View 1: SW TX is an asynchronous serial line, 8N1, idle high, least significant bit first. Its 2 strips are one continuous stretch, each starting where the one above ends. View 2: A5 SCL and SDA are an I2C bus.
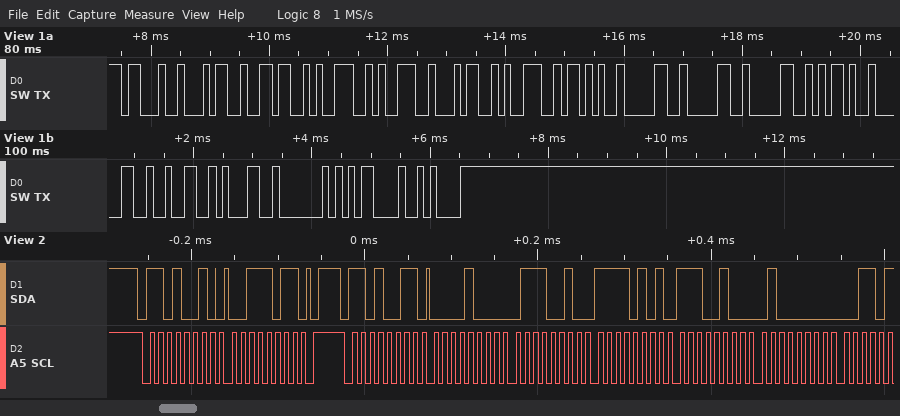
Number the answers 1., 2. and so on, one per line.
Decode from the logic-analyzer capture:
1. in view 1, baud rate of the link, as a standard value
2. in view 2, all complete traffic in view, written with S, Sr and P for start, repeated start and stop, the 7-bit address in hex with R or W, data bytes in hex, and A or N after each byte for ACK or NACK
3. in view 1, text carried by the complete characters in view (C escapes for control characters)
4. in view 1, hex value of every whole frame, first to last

1. 9600 baud
2. S 69W A 3B A P S 69R A 08 A 72 A F5 A E4 A 40 A
3. "#469949+000-021@\r\n"
4. 23 34 36 39 39 34 39 2B 30 30 30 2D 30 32 31 40 0D 0A
